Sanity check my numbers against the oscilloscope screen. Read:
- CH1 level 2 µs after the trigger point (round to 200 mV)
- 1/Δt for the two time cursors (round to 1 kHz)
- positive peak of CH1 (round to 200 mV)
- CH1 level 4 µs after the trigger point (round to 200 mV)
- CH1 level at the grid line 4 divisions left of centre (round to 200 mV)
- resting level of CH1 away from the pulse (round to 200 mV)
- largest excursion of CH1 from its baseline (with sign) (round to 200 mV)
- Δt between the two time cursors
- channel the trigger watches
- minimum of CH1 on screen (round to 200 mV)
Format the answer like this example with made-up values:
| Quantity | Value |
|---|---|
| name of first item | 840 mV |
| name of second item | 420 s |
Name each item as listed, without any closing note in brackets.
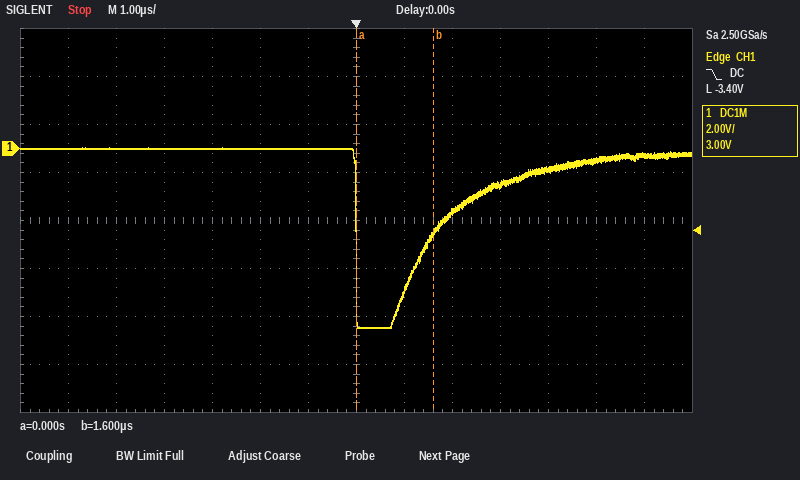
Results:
| Quantity | Value |
|---|---|
| CH1 level 2 µs after the trigger point | -2.6 V |
| 1/Δt for the two time cursors | 625 kHz |
| positive peak of CH1 | 0.0 V |
| CH1 level 4 µs after the trigger point | -800 mV |
| CH1 level at the grid line 4 divisions left of centre | 0.0 V |
| resting level of CH1 away from the pulse | 0.0 V |
| largest excursion of CH1 from its baseline (with sign) | -7.4 V |
| Δt between the two time cursors | 1.6 µs |
| channel the trigger watches | CH1 |
| minimum of CH1 on screen | -7.4 V |
